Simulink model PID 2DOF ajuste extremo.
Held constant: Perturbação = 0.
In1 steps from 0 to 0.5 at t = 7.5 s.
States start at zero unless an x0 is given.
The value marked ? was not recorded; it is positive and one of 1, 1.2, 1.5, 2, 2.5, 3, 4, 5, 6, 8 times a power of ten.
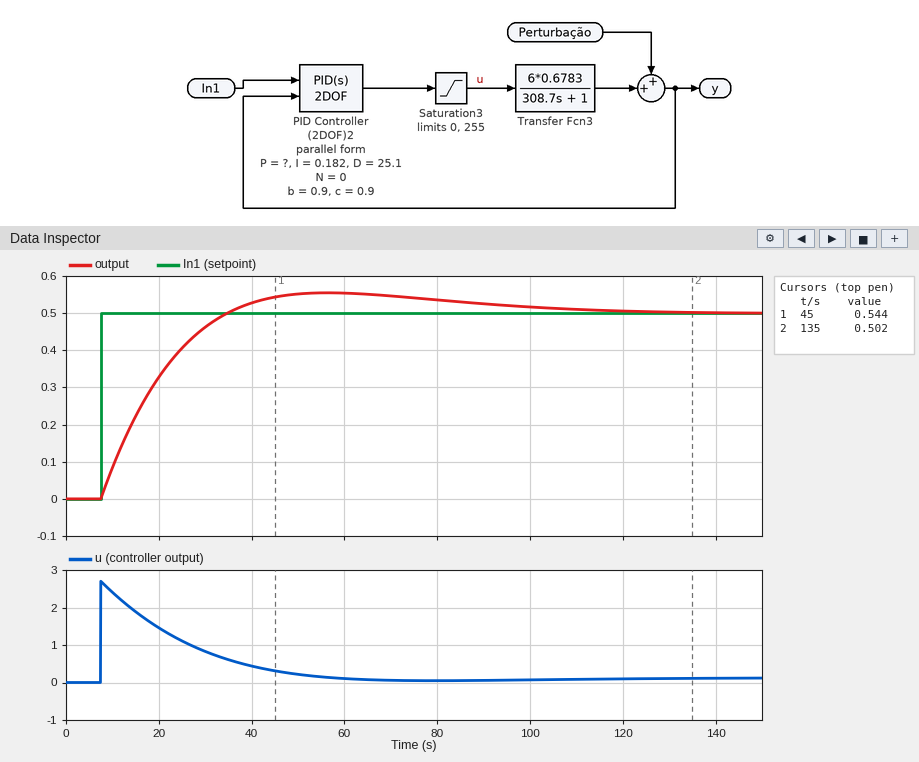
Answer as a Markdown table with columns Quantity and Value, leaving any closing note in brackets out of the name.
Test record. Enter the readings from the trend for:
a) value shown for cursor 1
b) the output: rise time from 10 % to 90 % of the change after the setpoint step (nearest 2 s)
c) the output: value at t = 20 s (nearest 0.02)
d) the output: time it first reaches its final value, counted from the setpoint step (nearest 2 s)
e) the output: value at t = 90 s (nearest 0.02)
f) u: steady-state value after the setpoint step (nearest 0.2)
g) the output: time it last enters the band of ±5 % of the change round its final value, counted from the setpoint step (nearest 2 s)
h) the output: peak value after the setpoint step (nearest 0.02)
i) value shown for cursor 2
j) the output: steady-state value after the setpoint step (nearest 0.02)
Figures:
| Quantity | Value |
|---|---|
| value shown for cursor 1 | 0.544 |
| the output: rise time from 10 % to 90 % of the change after the setpoint step | 20 s |
| the output: value at t = 20 s | 0.32 |
| the output: time it first reaches its final value, counted from the setpoint step | 28 s |
| the output: value at t = 90 s | 0.52 |
| u: steady-state value after the setpoint step | 0.2 |
| the output: time it last enters the band of ±5 % of the change round its final value, counted from the setpoint step | 82 s |
| the output: peak value after the setpoint step | 0.56 |
| value shown for cursor 2 | 0.502 |
| the output: steady-state value after the setpoint step | 0.50 |
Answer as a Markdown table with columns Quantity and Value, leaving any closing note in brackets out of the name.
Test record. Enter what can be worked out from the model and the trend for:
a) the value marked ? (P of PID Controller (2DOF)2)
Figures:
| Quantity | Value |
|---|---|
| the value marked ? (P of PID Controller (2DOF)2) | 6 |
